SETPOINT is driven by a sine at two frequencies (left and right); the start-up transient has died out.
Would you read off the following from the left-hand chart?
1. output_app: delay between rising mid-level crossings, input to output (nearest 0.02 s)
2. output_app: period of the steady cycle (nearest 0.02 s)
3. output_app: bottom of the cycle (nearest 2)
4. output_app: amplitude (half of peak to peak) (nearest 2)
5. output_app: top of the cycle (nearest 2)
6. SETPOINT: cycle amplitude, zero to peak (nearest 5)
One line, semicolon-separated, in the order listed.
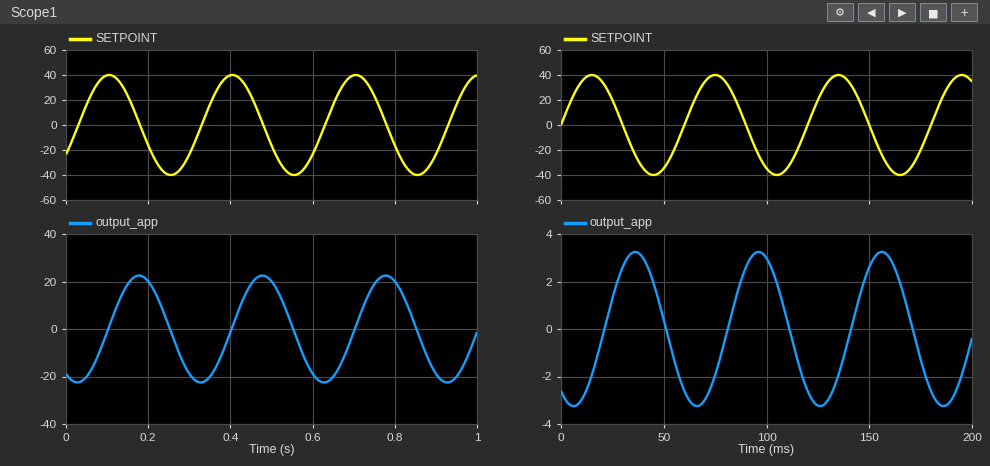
0.08 s; 0.30 s; -22; 22; 22; 40
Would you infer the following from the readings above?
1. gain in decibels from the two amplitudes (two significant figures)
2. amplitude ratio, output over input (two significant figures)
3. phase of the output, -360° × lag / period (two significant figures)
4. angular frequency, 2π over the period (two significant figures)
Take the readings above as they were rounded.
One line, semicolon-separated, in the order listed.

-5.2 dB; 0.55; -96°; 21 rad/s
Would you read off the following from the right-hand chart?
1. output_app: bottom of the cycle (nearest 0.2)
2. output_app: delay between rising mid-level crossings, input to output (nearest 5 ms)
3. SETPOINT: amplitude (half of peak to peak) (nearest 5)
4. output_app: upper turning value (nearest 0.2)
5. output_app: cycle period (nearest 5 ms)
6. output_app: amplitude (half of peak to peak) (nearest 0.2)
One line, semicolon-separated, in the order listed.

-3.2; 20 ms; 40; 3.2; 60 ms; 3.2
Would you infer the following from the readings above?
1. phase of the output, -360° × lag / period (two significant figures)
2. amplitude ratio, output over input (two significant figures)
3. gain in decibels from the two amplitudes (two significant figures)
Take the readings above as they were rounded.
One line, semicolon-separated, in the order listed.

-120°; 0.080; -22 dB
